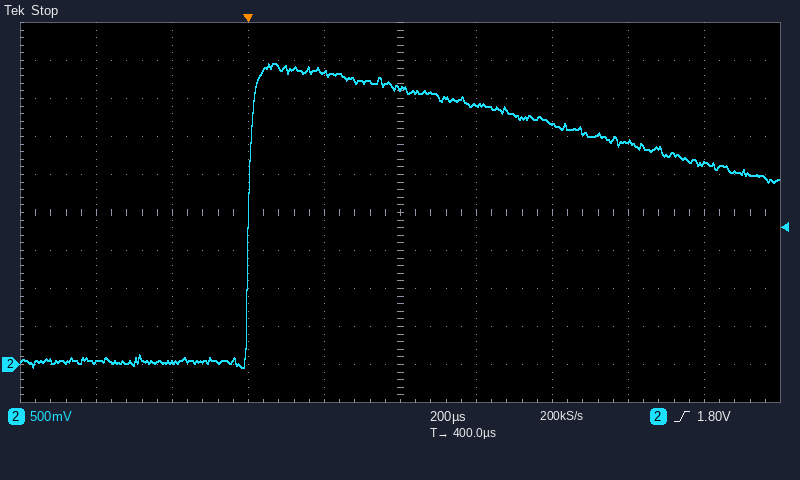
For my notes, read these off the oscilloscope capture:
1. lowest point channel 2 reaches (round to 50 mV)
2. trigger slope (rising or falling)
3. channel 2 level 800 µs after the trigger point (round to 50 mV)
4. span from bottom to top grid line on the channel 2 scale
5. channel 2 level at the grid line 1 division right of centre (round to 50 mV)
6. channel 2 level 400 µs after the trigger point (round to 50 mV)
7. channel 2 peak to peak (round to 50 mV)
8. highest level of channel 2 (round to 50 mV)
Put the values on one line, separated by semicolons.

-50 mV; rising; 3.15 V; 5 V; 3.40 V; 3.65 V; 4.00 V; 3.95 V
